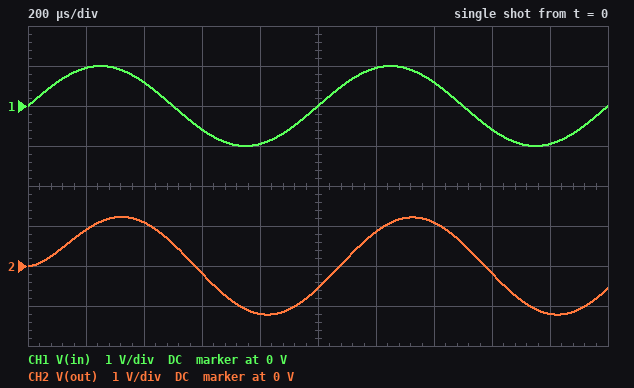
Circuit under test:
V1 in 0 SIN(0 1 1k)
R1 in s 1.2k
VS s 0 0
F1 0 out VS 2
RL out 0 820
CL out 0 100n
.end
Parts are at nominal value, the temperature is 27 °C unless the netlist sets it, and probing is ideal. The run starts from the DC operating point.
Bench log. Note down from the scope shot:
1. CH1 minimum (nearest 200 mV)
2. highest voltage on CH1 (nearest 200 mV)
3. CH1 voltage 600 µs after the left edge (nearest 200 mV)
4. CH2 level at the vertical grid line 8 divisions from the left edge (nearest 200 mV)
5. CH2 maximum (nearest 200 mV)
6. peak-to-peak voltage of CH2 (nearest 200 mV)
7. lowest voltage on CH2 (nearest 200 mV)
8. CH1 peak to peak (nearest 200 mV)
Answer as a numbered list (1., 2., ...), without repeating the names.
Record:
1. -1.0 V
2. 1.0 V
3. -600 mV
4. -200 mV
5. 1.2 V
6. 2.4 V
7. -1.2 V
8. 2.0 V
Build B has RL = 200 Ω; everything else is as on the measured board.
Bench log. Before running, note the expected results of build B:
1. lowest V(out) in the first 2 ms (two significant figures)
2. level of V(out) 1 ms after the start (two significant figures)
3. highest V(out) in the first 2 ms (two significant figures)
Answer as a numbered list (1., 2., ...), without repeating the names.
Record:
1. -330 mV
2. -41 mV
3. 330 mV
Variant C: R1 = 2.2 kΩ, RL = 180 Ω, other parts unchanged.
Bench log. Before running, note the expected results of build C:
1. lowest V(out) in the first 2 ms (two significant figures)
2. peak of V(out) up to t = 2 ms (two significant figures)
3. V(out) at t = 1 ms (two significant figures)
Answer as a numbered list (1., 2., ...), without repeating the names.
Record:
1. -160 mV
2. 160 mV
3. -18 mV
